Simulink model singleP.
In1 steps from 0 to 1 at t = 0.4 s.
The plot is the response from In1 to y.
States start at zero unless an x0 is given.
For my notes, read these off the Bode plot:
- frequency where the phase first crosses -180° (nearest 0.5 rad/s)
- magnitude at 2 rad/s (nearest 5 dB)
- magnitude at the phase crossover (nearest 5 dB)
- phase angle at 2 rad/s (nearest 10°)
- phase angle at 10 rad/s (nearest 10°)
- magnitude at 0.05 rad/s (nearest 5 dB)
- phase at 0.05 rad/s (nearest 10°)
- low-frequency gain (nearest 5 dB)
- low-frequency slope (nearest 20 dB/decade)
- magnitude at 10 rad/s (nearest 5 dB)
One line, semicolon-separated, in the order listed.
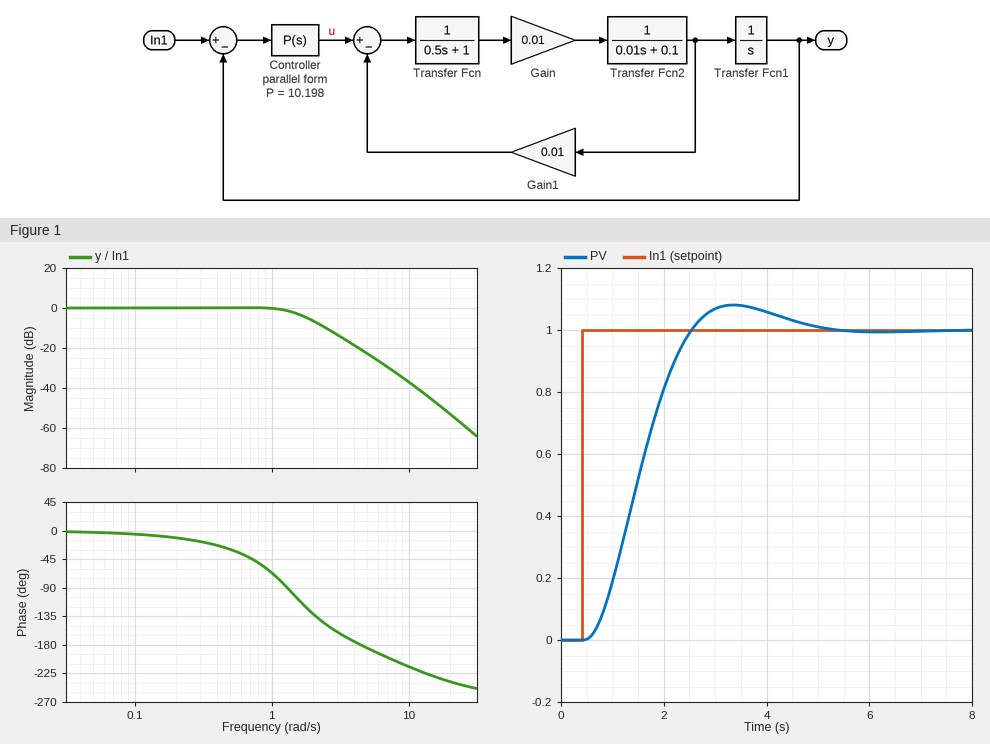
4.5 rad/s; -5 dB; -20 dB; -130°; -210°; 0 dB; 0°; 0 dB; 0 dB/decade; -35 dB
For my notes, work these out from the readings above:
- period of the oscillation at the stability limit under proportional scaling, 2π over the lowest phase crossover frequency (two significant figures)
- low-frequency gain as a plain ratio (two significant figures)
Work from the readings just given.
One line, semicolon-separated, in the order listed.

1.4 s; 1.0
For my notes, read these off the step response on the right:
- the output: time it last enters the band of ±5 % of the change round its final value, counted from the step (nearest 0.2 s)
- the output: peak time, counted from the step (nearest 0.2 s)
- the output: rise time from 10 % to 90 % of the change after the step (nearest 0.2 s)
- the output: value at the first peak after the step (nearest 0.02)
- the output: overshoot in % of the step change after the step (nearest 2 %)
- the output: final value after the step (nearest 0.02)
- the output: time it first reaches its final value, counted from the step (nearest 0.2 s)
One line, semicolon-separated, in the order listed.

3.8 s; 3.0 s; 1.4 s; 1.08; 8 %; 1.00; 2.2 s
